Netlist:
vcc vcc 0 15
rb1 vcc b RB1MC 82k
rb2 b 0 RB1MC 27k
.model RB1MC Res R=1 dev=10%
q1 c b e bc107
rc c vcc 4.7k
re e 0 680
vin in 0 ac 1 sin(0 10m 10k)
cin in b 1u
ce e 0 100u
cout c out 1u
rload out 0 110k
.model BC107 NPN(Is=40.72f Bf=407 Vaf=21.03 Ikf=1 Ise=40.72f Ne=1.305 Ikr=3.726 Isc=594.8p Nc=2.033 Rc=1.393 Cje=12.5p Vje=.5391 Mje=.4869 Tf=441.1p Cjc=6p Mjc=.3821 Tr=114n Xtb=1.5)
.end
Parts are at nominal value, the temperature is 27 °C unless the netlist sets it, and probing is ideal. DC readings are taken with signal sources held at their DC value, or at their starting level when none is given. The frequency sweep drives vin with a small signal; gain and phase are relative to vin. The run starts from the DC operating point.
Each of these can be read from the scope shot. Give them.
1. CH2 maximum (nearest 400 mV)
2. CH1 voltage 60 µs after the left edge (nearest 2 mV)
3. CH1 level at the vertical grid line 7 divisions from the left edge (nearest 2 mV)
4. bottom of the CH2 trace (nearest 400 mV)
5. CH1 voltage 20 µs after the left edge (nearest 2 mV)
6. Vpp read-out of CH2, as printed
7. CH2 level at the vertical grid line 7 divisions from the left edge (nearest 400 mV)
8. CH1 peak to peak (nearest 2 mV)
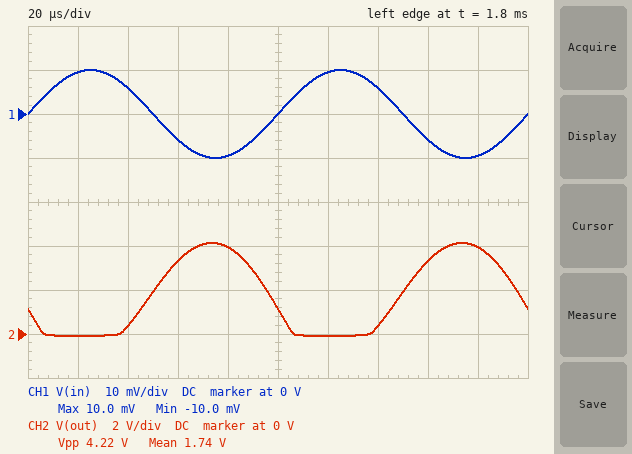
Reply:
4.0 V
-6 mV
6 mV
0 V
10 mV
4.22 V
400 mV
20 mV
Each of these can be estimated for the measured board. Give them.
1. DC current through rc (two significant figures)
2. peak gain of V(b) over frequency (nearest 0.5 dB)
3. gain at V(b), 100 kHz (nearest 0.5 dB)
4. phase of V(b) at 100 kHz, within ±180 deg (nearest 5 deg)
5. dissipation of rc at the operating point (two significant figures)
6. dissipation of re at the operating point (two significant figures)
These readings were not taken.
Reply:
2.8 mA
0 dB
0 dB
5 deg
36 mW
5.4 mW
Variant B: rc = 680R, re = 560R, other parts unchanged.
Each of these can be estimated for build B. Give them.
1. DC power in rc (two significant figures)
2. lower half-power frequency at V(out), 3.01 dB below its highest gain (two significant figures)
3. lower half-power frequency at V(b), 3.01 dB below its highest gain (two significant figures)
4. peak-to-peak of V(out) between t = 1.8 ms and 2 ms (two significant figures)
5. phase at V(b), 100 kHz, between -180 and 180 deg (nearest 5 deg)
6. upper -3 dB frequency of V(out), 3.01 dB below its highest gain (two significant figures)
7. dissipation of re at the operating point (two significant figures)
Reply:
16 mW
370 Hz
24 Hz
2.2 V
0 deg
110 MHz
13 mW
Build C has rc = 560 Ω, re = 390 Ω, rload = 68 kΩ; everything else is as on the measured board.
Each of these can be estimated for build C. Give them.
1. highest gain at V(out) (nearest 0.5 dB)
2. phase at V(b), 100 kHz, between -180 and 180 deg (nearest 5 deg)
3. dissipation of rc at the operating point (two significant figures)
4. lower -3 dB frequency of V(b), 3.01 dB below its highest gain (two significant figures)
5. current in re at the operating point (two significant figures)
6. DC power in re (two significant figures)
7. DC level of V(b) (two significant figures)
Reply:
42.0 dB
0 deg
24 mW
24 Hz
6.6 mA
17 mW
3.2 V
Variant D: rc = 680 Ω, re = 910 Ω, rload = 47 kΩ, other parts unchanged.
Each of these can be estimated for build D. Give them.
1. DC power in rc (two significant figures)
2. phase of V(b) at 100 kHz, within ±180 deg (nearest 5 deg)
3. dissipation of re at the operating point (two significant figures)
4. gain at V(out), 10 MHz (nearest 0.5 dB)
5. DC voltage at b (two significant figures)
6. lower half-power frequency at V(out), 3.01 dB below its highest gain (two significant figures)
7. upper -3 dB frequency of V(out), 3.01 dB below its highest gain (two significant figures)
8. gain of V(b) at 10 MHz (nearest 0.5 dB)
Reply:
6.5 mW
0 deg
8.8 mW
37.5 dB
3.5 V
250 Hz
110 MHz
0 dB
